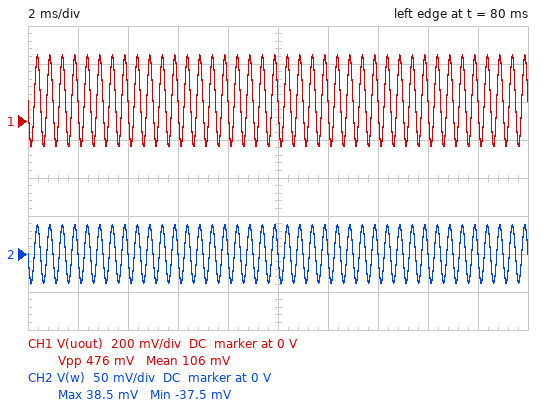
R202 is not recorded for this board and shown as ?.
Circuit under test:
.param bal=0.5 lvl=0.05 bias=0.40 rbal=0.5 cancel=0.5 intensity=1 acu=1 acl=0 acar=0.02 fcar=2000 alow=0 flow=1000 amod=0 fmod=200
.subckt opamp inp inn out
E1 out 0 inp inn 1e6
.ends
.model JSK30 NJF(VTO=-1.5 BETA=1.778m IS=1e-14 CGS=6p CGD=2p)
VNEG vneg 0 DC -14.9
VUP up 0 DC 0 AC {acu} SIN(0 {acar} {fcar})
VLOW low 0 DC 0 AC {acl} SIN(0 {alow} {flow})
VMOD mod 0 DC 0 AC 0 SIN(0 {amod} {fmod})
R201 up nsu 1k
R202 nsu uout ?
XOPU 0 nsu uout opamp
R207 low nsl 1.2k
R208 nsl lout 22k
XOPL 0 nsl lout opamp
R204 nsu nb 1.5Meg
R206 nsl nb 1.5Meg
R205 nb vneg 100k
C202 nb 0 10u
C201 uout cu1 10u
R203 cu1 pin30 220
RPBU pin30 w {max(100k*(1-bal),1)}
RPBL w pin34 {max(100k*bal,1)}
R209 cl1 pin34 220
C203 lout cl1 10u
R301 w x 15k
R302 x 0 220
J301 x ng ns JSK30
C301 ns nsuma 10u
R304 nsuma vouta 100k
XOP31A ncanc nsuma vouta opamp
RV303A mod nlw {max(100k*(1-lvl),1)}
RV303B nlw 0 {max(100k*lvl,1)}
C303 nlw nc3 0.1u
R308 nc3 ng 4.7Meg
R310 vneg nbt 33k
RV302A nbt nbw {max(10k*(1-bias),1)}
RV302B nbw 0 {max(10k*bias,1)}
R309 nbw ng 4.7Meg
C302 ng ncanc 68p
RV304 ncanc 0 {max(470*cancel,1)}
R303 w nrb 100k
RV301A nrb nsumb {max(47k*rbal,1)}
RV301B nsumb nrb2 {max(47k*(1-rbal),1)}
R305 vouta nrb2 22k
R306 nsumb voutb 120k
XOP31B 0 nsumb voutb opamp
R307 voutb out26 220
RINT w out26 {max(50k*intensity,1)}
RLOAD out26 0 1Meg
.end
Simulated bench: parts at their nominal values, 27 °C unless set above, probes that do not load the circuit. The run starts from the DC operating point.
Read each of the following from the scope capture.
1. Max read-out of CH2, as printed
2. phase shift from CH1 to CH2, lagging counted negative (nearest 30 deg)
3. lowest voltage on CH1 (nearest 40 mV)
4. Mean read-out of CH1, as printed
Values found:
38.5 mV
0 deg
-120 mV
106 mV
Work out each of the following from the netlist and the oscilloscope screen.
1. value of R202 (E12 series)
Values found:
12 kΩ
